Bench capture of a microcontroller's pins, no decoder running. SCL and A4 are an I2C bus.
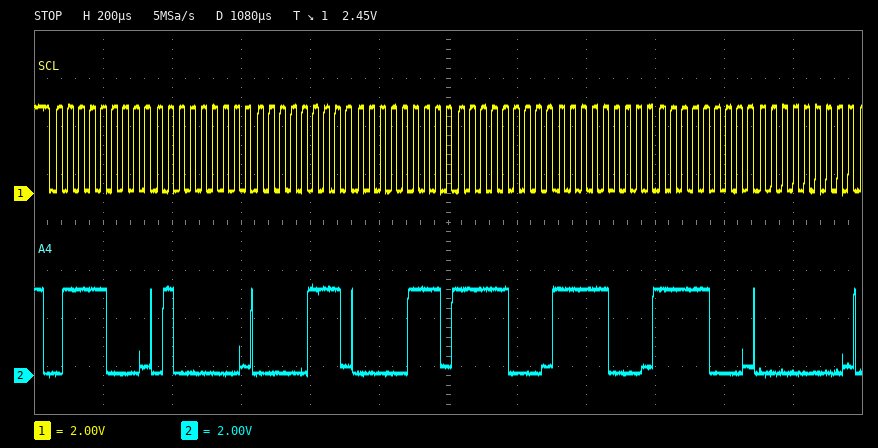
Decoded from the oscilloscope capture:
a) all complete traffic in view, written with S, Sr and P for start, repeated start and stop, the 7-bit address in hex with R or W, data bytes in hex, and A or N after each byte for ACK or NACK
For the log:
S 3CW A 40 A 07 A 07 A F8 A F8 A F8 A 00 A
